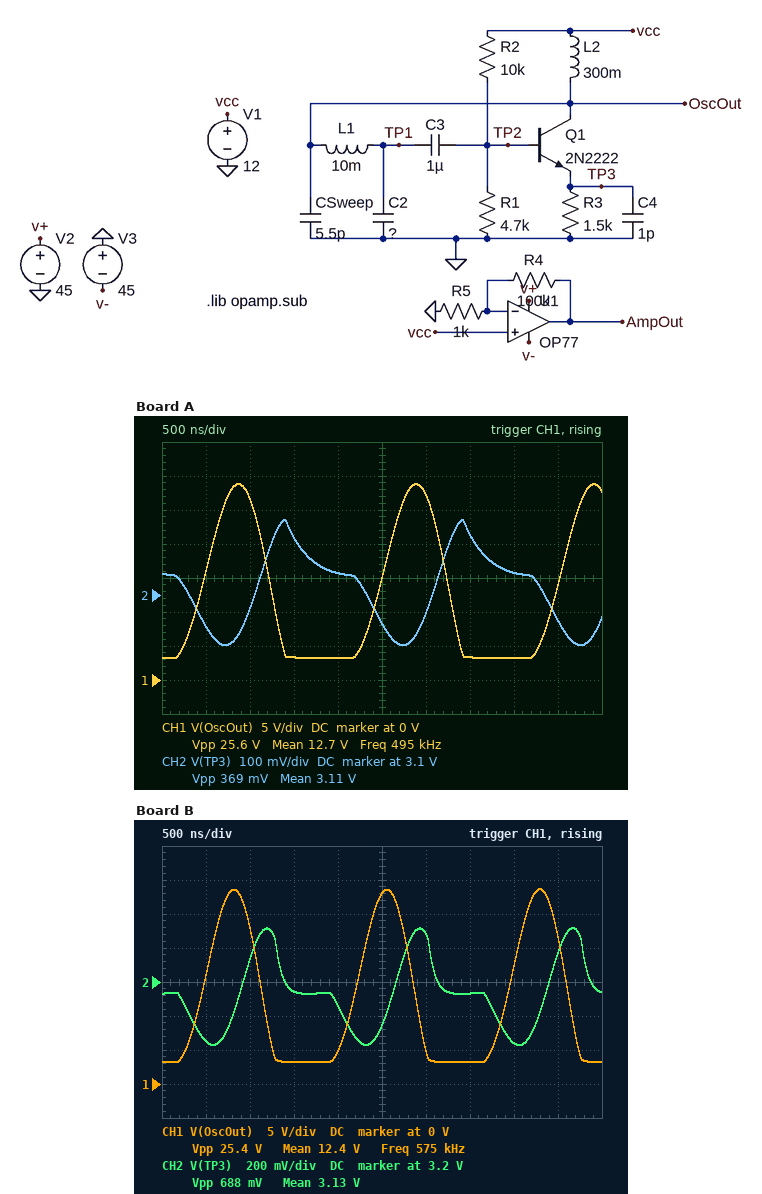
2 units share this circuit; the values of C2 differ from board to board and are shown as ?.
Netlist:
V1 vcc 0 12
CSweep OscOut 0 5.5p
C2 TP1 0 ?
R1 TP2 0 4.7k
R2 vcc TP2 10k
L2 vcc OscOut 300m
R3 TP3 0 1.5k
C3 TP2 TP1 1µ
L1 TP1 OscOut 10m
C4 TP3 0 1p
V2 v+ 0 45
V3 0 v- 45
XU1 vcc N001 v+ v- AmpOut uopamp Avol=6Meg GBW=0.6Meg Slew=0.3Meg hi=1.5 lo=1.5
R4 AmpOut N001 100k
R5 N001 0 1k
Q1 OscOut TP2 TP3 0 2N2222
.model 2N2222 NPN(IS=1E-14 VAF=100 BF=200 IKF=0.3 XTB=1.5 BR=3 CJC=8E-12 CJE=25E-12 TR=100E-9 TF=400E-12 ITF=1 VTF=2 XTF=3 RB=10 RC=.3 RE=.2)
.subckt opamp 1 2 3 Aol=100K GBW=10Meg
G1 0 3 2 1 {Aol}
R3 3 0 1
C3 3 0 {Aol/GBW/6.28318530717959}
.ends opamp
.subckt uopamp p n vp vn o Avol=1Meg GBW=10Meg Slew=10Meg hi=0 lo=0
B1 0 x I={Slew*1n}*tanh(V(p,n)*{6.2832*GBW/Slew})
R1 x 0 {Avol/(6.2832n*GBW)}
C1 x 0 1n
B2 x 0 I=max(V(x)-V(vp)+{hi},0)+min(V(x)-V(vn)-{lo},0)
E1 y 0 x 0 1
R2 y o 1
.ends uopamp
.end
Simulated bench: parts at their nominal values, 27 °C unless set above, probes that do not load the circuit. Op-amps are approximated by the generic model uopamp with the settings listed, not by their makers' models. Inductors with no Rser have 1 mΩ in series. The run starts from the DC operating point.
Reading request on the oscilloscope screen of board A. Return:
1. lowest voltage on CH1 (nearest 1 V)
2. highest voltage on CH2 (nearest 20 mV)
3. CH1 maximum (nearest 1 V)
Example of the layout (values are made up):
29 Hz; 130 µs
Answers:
3 V; 3.32 V; 29 V
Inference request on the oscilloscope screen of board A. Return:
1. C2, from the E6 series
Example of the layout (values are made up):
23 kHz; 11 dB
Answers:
330 pF
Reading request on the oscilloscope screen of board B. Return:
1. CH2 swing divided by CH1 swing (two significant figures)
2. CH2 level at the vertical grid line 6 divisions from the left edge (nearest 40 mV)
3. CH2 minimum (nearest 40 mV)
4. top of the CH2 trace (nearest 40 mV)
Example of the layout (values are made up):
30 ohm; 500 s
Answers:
0.027; 3.48 V; 2.84 V; 3.52 V
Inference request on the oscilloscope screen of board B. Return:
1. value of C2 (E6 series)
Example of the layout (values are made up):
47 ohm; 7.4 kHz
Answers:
68 pF
